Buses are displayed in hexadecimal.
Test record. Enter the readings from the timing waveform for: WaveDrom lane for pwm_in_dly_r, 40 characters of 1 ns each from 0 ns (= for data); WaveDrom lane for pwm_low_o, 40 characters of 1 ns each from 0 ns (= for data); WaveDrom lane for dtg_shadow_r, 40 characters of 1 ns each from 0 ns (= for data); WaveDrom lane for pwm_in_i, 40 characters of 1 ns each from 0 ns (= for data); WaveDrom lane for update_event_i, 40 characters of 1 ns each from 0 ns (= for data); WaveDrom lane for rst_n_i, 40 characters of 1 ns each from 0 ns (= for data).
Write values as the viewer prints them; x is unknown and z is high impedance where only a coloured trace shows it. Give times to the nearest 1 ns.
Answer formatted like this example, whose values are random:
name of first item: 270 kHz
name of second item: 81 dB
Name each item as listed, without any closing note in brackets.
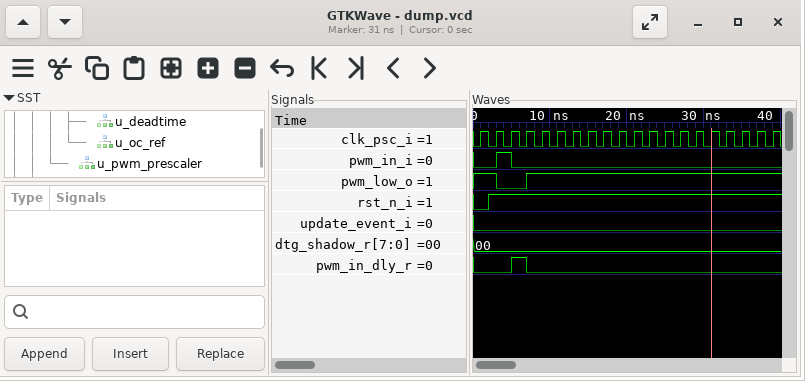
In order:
WaveDrom lane for pwm_in_dly_r, 40 characters of 1 ns each from 0 ns: {name: 'pwm_in_dly_r', wave: '0....1.0................................'}
WaveDrom lane for pwm_low_o, 40 characters of 1 ns each from 0 ns: {name: 'pwm_low_o', wave: '1..0...1................................'}
WaveDrom lane for dtg_shadow_r, 40 characters of 1 ns each from 0 ns: {name: 'dtg_shadow_r', wave: '=.......................................', data: '00'}
WaveDrom lane for pwm_in_i, 40 characters of 1 ns each from 0 ns: {name: 'pwm_in_i', wave: '0..1.0..................................'}
WaveDrom lane for update_event_i, 40 characters of 1 ns each from 0 ns: {name: 'update_event_i', wave: '0.......................................'}
WaveDrom lane for rst_n_i, 40 characters of 1 ns each from 0 ns: {name: 'rst_n_i', wave: '0.1.....................................'}
